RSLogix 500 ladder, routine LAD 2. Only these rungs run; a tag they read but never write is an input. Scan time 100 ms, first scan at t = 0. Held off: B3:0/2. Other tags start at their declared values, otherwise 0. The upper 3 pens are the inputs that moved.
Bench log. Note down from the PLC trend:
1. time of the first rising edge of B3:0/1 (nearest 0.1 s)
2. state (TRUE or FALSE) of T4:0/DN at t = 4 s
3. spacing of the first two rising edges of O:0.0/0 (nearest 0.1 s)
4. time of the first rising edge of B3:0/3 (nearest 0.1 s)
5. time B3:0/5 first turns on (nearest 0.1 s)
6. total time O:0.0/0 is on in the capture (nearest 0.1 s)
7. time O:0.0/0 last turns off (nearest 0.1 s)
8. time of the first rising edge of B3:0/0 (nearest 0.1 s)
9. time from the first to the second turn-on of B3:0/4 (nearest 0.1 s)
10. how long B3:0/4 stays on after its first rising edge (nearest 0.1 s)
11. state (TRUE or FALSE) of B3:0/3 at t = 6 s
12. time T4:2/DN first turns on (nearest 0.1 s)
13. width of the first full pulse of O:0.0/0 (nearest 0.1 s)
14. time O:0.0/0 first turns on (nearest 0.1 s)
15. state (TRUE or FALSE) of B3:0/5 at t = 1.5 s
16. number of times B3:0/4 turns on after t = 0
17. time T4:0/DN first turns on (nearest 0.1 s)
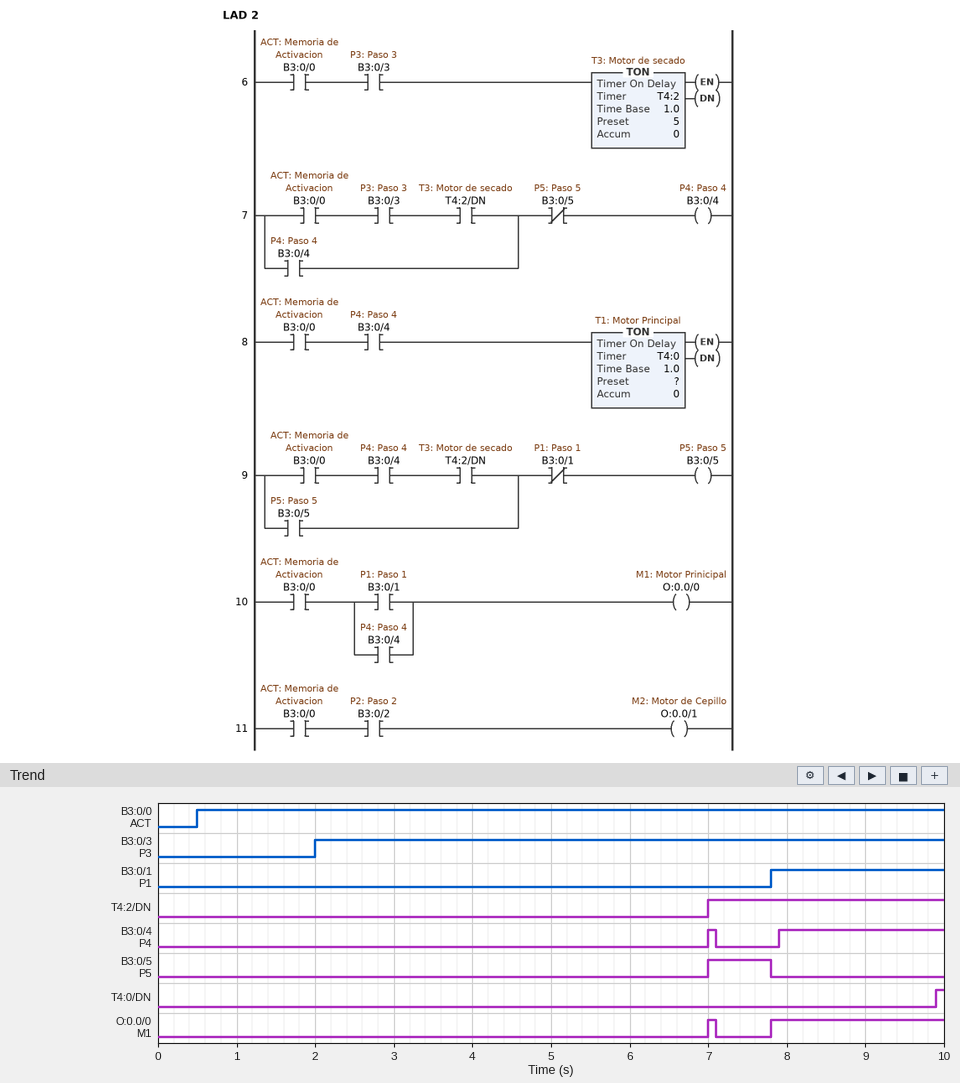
7.8 s
FALSE
0.8 s
2.0 s
7.0 s
2.3 s
7.1 s
0.5 s
0.9 s
0.1 s
TRUE
7.0 s
0.1 s
7.0 s
FALSE
2
9.9 s
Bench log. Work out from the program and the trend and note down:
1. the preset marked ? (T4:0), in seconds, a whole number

2 s
